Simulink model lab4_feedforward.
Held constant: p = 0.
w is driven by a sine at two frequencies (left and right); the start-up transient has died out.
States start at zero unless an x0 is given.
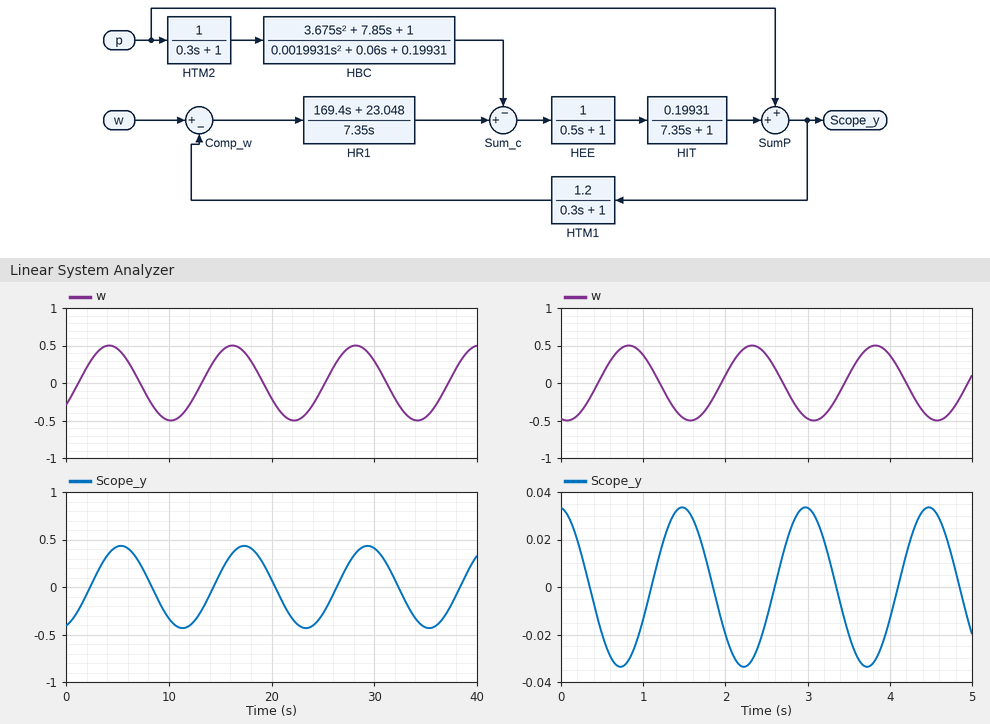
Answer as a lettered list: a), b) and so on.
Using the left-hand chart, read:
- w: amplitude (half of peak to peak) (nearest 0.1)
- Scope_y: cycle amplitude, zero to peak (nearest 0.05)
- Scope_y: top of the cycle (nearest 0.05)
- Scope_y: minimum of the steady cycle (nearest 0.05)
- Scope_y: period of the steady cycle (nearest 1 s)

a) 0.5
b) 0.45
c) 0.45
d) -0.45
e) 12 s
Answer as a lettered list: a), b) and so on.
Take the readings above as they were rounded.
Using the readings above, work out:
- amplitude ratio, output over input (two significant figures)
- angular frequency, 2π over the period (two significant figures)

a) 0.90
b) 0.52 rad/s
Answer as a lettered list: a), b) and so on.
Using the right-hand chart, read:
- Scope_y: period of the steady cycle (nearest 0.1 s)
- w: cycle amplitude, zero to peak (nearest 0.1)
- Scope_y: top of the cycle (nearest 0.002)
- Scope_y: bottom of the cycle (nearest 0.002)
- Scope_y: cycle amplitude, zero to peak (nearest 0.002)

a) 1.5 s
b) 0.5
c) 0.034
d) -0.034
e) 0.034
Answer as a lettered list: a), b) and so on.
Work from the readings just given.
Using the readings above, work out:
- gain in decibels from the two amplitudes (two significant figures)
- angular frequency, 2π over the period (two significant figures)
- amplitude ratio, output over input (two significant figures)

a) -23 dB
b) 4.2 rad/s
c) 0.068
